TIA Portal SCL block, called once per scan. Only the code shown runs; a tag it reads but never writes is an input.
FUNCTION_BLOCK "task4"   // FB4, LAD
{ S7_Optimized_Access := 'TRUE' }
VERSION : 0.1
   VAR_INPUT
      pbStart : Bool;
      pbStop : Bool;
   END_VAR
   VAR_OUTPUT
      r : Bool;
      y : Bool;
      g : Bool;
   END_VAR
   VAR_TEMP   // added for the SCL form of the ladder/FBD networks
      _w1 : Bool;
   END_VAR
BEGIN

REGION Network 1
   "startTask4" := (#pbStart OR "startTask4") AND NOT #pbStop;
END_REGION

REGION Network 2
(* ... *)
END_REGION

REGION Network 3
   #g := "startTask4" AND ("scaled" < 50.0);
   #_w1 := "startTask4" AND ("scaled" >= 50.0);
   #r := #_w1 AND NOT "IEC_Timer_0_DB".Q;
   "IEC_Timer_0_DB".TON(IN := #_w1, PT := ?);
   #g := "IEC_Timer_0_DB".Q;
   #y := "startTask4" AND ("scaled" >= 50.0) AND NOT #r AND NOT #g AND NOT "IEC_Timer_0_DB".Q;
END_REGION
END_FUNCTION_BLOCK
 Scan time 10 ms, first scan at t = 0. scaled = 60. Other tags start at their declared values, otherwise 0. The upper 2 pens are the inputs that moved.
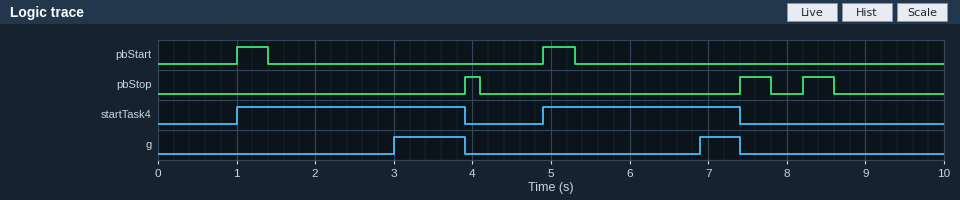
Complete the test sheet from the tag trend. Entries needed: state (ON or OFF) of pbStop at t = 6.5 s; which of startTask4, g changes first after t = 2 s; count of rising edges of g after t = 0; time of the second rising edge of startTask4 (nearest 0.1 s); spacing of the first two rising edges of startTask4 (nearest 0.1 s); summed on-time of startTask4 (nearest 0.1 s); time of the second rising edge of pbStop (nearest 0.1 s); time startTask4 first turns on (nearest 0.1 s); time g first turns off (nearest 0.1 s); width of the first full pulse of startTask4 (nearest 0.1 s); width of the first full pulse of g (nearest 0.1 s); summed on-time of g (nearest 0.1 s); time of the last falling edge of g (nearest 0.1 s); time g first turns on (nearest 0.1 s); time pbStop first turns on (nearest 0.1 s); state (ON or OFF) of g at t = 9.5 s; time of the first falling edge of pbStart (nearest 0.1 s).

OFF
g
2
4.9 s
3.9 s
5.4 s
7.4 s
1.0 s
3.9 s
2.9 s
0.9 s
1.4 s
7.4 s
3.0 s
3.9 s
OFF
1.4 s
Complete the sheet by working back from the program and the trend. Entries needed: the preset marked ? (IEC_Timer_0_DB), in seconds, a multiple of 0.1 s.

2.0 s
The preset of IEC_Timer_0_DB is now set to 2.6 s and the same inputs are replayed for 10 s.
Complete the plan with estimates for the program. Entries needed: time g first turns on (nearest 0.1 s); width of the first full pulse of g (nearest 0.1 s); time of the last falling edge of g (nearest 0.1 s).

3.6 s
0.3 s
3.9 s
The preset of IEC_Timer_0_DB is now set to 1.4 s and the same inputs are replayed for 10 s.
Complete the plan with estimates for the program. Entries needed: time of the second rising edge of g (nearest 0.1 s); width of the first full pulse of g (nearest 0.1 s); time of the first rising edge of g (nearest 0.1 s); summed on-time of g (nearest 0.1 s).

6.3 s
1.5 s
2.4 s
2.6 s
